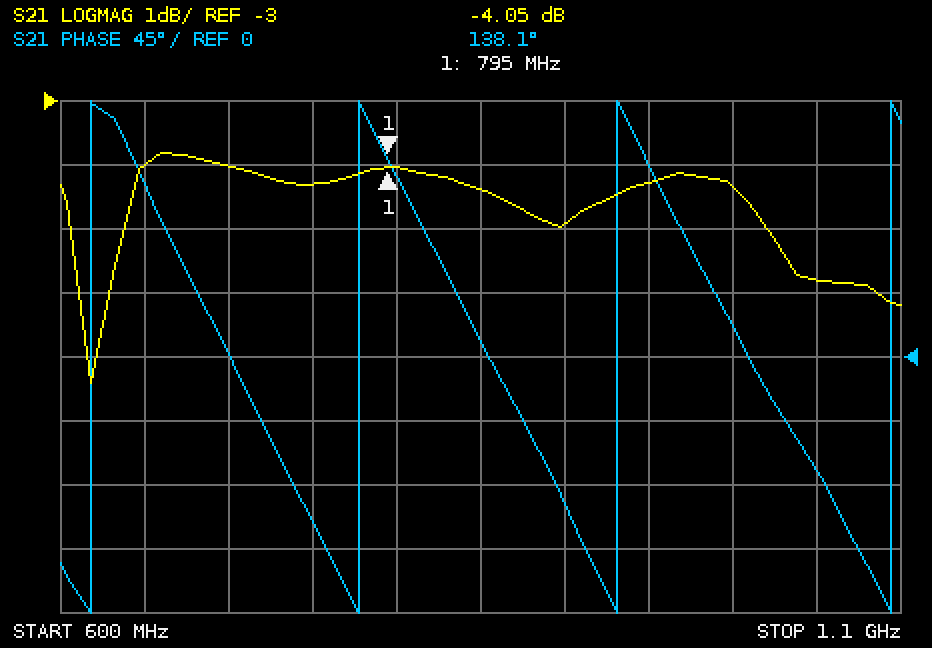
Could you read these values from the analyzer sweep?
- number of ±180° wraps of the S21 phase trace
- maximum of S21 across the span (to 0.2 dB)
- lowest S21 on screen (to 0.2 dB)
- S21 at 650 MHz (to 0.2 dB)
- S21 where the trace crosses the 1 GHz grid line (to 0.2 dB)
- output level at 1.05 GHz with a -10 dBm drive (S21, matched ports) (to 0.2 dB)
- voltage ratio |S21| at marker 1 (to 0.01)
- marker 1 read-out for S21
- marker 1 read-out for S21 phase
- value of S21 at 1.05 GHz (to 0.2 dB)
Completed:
4
-3.8 dB
-7.4 dB
-4.0 dB
-4.4 dB
-15.8 dBm
0.63
-4.05 dB
138.1°
-5.8 dB
